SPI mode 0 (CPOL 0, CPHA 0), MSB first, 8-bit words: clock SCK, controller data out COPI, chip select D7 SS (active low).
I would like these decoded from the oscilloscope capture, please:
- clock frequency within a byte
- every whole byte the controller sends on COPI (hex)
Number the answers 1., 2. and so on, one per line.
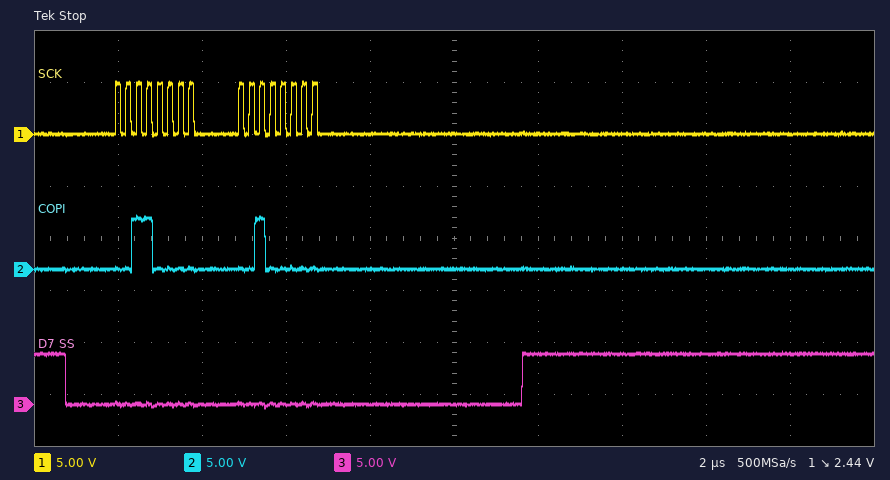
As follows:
1. 4 MHz
2. 30 20
